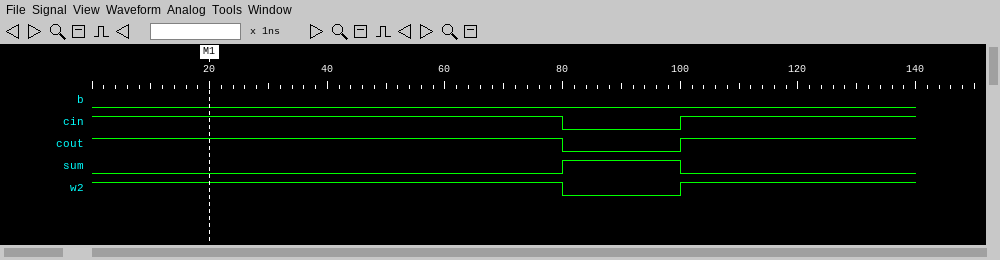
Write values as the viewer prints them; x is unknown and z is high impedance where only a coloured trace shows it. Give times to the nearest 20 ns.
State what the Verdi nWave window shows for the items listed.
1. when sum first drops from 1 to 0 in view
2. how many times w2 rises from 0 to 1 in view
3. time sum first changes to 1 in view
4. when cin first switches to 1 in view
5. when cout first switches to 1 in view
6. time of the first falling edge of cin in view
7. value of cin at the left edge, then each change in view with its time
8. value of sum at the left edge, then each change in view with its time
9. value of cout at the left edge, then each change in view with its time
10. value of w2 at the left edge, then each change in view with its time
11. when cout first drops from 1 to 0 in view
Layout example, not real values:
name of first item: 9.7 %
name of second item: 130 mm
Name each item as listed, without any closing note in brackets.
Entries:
when sum first drops from 1 to 0 in view: 100 ns
how many times w2 rises from 0 to 1 in view: 1
time sum first changes to 1 in view: 80 ns
when cin first switches to 1 in view: 100 ns
when cout first switches to 1 in view: 100 ns
time of the first falling edge of cin in view: 80 ns
value of cin at the left edge, then each change in view with its time: 1, 0 at 80 ns, 1 at 100 ns
value of sum at the left edge, then each change in view with its time: 0, 1 at 80 ns, 0 at 100 ns
value of cout at the left edge, then each change in view with its time: 1, 0 at 80 ns, 1 at 100 ns
value of w2 at the left edge, then each change in view with its time: 1, 0 at 80 ns, 1 at 100 ns
when cout first drops from 1 to 0 in view: 80 ns
